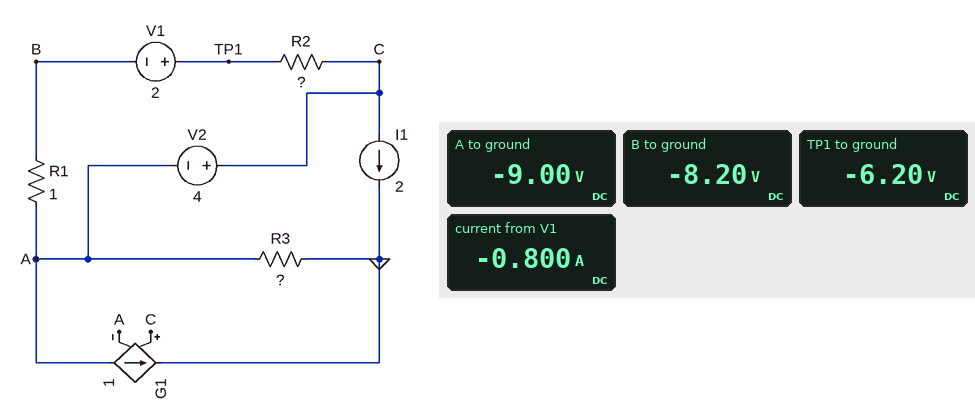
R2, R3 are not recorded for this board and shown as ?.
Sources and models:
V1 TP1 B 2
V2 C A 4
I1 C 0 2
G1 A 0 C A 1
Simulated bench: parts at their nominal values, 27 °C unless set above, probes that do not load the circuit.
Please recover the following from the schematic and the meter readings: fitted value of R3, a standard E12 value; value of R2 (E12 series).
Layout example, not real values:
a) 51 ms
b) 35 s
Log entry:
a) 1.5 Ω
b) 1.5 Ω
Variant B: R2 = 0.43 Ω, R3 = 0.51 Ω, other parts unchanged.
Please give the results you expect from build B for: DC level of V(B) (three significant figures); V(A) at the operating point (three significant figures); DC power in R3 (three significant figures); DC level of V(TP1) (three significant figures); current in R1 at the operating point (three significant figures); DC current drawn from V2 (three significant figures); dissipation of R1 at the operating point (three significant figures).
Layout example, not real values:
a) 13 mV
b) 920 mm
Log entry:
a) -1.66 V
b) -3.06 V
c) 18.4 W
d) 339 mV
e) 1.40 A
f) 3.40 A
g) 1.96 W
